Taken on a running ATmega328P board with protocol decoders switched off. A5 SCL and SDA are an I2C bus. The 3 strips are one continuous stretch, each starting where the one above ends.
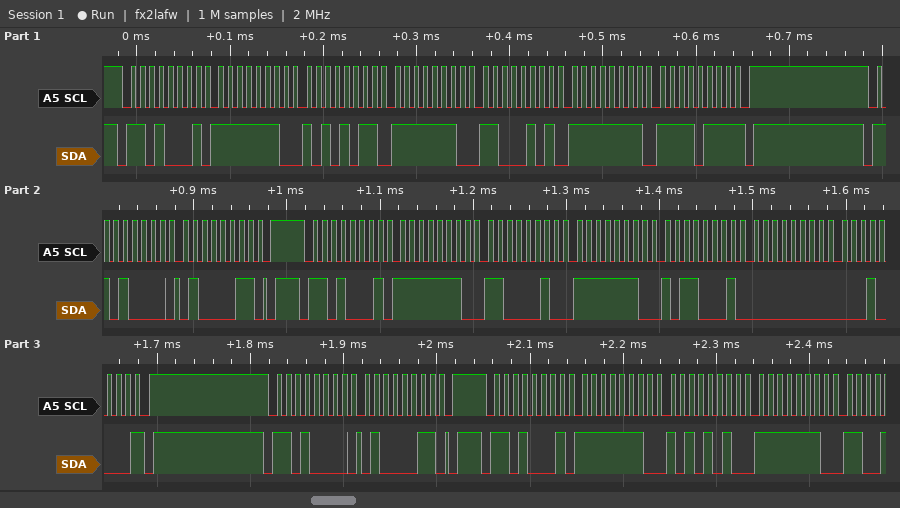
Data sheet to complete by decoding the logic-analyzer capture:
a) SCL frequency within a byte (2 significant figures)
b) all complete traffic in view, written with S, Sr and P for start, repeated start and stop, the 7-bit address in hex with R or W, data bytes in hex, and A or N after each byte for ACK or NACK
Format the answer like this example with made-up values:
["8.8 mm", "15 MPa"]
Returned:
["100 kHz", "S 68R A FE A AB A FE A C5 A FF A F7 N P S 68W A 43 A P S 68R A FE A C2 A FE A B1 A 00 A 10 N P S 68W A 43 A P S 68R A FE A AA A FE A"]
